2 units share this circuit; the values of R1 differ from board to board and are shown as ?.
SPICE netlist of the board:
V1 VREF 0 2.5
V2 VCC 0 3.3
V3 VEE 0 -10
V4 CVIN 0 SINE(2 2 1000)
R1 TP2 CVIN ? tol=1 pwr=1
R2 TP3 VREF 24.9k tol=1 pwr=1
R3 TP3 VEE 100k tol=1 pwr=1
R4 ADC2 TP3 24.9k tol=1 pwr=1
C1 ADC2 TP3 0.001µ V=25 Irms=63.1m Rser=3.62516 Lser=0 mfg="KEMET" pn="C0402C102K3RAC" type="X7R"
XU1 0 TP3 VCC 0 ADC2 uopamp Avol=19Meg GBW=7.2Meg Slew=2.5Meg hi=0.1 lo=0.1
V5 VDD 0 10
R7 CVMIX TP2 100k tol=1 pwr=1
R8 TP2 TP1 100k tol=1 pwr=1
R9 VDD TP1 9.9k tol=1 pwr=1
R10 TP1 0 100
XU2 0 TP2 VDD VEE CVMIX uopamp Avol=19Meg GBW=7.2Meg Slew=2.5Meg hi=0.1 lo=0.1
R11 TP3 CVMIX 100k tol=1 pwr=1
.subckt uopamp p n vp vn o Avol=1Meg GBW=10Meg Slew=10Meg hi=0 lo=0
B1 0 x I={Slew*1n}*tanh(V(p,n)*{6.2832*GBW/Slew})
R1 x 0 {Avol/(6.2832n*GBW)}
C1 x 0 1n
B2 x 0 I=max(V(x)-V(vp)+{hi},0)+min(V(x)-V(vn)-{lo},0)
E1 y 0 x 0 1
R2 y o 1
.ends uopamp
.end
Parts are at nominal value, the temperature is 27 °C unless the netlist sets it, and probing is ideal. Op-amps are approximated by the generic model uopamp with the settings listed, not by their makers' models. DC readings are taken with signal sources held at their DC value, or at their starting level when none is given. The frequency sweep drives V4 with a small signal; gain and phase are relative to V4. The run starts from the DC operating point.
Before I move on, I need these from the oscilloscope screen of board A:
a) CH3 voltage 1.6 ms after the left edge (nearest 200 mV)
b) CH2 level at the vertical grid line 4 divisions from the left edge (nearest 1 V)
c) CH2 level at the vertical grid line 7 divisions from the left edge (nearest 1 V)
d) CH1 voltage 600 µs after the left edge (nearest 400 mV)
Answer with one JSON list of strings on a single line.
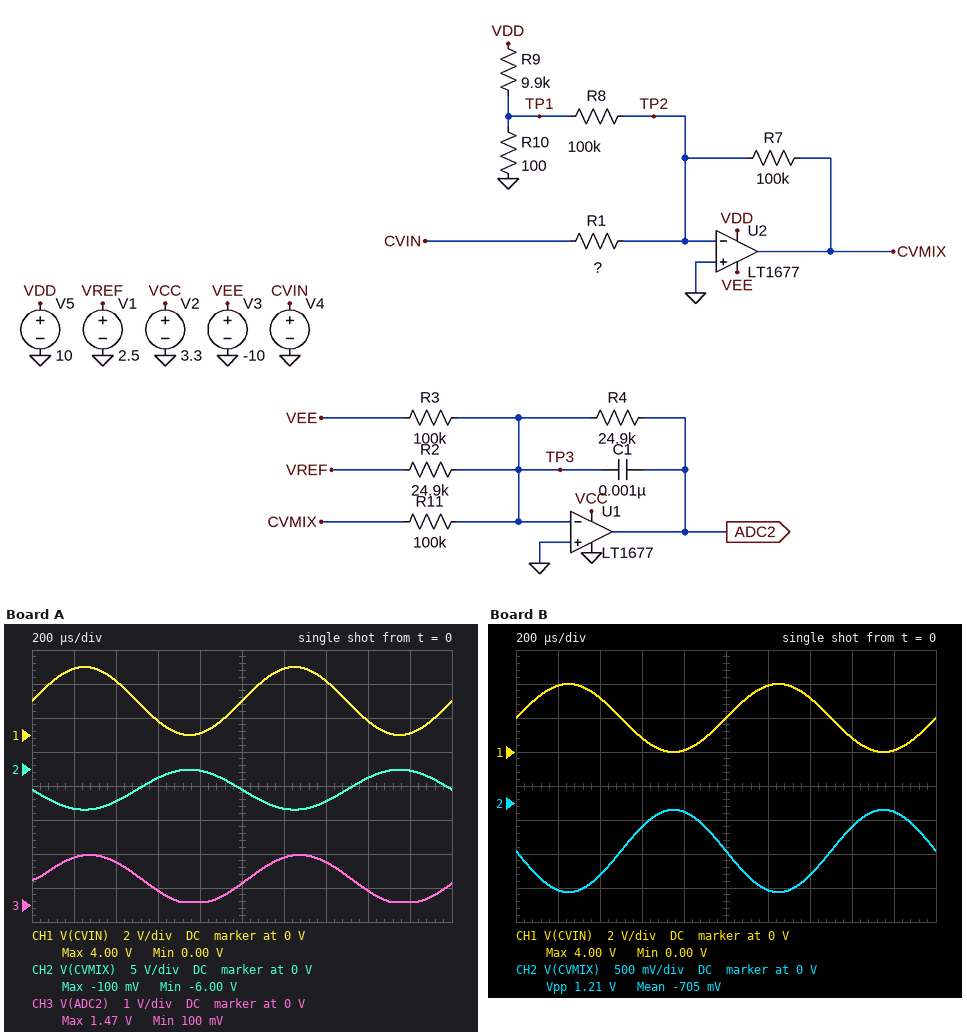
["400 mV", "0 V", "-5 V", "800 mV"]
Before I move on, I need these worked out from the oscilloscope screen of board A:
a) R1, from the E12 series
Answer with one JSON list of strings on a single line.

["68 kΩ"]
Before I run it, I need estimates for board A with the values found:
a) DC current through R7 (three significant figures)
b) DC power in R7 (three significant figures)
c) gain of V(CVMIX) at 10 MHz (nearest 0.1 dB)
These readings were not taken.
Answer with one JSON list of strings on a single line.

["30.4 µA", "92.5 µW", "-10.5 dB"]
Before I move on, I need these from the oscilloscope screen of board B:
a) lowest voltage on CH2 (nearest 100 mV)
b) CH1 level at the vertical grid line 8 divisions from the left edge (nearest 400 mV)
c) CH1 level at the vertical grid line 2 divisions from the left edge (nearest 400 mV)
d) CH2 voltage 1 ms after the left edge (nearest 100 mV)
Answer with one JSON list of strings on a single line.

["-1.3 V", "800 mV", "3.2 V", "-700 mV"]
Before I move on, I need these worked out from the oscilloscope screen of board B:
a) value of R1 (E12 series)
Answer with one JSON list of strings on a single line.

["330 kΩ"]
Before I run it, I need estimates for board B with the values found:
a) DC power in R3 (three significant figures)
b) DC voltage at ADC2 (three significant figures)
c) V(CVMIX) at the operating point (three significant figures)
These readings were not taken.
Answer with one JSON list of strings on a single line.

["1.00 mW", "166 mV", "-706 mV"]
